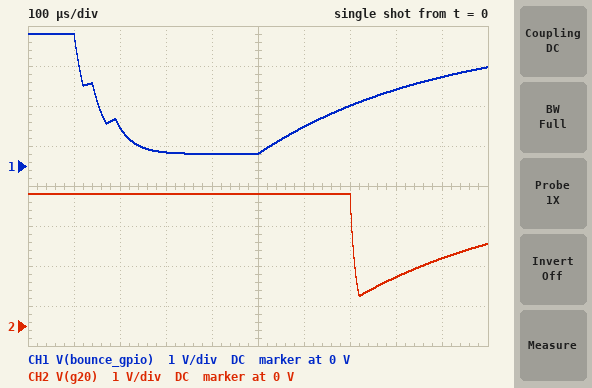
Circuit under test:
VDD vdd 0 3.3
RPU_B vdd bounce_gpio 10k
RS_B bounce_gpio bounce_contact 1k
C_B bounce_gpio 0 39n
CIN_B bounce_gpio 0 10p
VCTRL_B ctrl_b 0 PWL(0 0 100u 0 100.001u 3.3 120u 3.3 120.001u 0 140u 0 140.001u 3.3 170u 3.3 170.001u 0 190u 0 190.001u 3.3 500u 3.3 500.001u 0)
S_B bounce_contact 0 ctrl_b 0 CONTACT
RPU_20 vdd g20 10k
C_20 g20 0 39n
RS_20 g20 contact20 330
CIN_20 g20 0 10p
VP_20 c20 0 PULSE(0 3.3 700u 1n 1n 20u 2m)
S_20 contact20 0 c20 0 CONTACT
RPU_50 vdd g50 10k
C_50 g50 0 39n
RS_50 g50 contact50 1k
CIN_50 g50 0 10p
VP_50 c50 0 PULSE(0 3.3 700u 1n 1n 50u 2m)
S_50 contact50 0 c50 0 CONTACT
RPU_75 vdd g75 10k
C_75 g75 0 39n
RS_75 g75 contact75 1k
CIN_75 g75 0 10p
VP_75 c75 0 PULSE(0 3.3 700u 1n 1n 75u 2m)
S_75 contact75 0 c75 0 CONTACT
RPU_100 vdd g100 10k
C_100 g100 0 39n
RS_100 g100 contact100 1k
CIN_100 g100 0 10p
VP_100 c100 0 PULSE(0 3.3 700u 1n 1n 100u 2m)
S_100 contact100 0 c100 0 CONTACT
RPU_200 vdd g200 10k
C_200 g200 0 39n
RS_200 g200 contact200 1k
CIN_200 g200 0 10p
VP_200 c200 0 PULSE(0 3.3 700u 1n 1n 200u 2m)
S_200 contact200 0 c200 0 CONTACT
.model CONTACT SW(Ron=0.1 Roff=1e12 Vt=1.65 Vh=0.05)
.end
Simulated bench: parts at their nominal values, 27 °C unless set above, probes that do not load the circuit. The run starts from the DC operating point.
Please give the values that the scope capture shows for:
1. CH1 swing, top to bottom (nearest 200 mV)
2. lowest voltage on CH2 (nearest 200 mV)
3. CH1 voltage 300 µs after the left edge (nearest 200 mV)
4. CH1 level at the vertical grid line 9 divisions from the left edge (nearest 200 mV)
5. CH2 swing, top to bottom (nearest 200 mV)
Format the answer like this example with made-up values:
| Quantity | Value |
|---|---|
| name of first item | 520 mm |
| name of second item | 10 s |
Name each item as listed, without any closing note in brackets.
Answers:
| Quantity | Value |
|---|---|
| CH1 swing, top to bottom | 3.0 V |
| lowest voltage on CH2 | 800 mV |
| CH1 voltage 300 µs after the left edge | 400 mV |
| CH1 level at the vertical grid line 9 divisions from the left edge | 2.2 V |
| CH2 swing, top to bottom | 2.6 V |
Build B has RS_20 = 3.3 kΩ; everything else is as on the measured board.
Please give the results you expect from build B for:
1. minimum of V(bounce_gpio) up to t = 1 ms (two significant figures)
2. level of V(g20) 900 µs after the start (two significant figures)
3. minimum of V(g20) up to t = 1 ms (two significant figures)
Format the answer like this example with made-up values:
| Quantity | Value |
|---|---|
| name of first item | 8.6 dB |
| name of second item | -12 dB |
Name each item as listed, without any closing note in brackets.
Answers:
| Quantity | Value |
|---|---|
| minimum of V(bounce_gpio) up to t = 1 ms | 300 mV |
| level of V(g20) 900 µs after the start | 3.0 V |
| minimum of V(g20) up to t = 1 ms | 2.8 V |
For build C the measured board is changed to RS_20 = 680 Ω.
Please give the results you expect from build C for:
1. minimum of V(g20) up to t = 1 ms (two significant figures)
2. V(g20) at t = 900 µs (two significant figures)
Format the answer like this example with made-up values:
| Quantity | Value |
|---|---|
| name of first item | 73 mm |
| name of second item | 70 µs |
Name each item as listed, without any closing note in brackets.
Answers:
| Quantity | Value |
|---|---|
| minimum of V(g20) up to t = 1 ms | 1.6 V |
| V(g20) at t = 900 µs | 2.2 V |
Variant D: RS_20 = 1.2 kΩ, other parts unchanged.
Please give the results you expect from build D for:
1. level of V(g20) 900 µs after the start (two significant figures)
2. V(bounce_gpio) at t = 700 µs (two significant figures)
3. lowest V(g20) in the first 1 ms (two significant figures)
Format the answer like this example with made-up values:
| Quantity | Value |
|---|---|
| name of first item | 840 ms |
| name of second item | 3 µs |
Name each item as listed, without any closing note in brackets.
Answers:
| Quantity | Value |
|---|---|
| level of V(g20) 900 µs after the start | 2.6 V |
| V(bounce_gpio) at t = 700 µs | 1.5 V |
| lowest V(g20) in the first 1 ms | 2.2 V |
